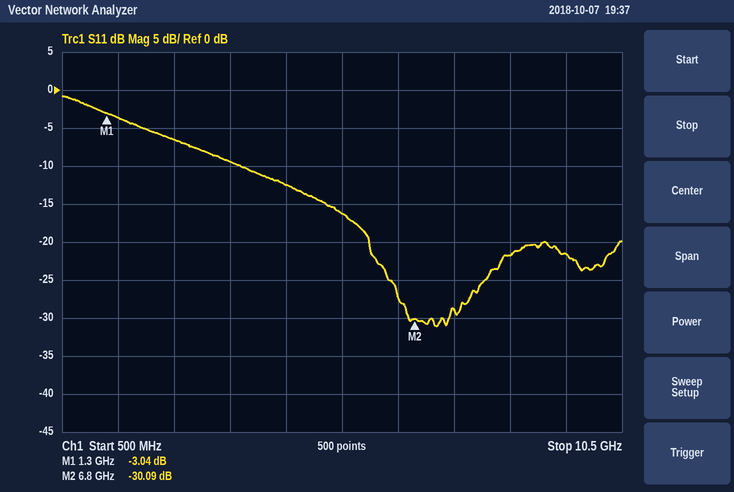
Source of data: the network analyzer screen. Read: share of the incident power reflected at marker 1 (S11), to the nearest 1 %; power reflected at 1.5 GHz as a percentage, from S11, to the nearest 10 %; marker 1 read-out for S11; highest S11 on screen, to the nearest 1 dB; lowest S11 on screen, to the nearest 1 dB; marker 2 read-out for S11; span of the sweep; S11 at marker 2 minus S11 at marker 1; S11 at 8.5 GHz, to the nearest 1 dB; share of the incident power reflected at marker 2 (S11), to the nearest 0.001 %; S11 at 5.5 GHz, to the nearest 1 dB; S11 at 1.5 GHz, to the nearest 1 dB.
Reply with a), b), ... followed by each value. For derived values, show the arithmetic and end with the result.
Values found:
a) 10^(-3.04/10) ≈ 50 %
b) 10^(-4/10) ≈ 40 %
c) -3.04 dB
d) -1 dB
e) -31 dB
f) -30.09 dB
g) 10 GHz
h) -30.09 − (-3.04) = -27.05 dB
i) -22 dB
j) 10^(-30.09/10) ≈ 0.098 %
k) -16 dB
l) -4 dB
